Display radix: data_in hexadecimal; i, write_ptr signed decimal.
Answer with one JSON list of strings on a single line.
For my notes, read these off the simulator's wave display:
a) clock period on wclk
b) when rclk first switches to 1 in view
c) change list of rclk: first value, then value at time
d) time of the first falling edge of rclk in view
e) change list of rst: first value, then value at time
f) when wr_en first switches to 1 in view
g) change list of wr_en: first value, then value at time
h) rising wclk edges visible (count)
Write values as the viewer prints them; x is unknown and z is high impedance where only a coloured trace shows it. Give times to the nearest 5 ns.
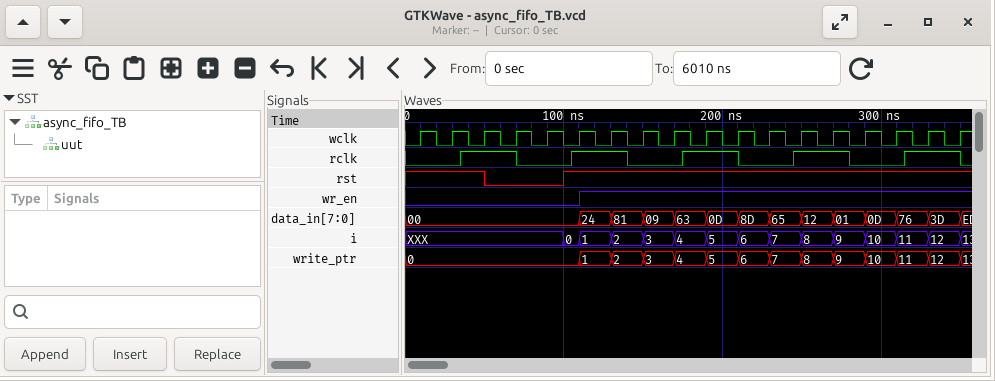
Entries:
["20 ns", "35 ns", "0, 1 at 35 ns, 0 at 70 ns, 1 at 105 ns, 0 at 140 ns, 1 at 175 ns, 0 at 210 ns, 1 at 245 ns, 0 at 280 ns, 1 at 315 ns, 0 at 350 ns", "70 ns", "1, 0 at 50 ns, 1 at 100 ns", "110 ns", "0, 1 at 110 ns", "18"]
